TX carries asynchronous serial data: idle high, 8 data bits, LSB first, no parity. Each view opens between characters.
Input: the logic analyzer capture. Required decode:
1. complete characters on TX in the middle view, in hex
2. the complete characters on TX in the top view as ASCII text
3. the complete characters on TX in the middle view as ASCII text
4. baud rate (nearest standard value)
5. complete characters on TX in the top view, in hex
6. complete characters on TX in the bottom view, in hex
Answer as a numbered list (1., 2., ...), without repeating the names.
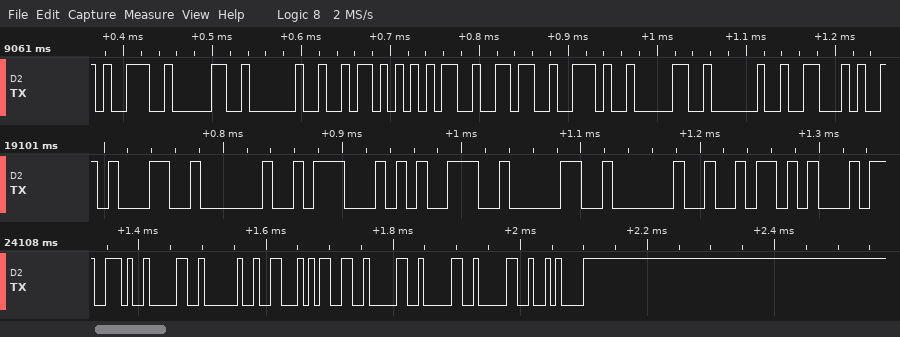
1. 31, 20, 47, 39, 30, 20, 5A
2. "90 Z56.0 F"
3. "1 G90 Z"
4. 115200 baud
5. 39, 30, 20, 5A, 35, 36, 2E, 30, 20, 46
6. 2E, 30, 20, 46, 33, 30, 30, 30, 0A
